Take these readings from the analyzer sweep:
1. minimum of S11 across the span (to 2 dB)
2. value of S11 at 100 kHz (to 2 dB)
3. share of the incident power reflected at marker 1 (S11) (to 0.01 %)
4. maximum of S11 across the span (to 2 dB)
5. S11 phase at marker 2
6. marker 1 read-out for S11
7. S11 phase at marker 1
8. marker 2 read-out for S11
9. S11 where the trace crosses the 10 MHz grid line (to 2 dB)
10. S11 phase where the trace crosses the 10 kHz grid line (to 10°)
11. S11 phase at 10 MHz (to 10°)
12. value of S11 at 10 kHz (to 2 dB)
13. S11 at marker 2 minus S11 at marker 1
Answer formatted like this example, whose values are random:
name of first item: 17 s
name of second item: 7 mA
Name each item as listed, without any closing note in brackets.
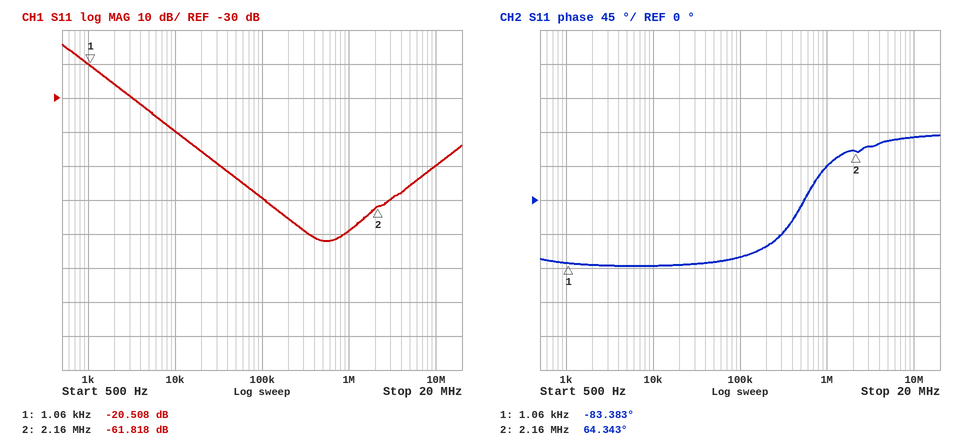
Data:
minimum of S11 across the span: -72 dB
value of S11 at 100 kHz: -60 dB
share of the incident power reflected at marker 1 (S11): 0.89 %
maximum of S11 across the span: -14 dB
S11 phase at marker 2: 64.343°
marker 1 read-out for S11: -20.508 dB
S11 phase at marker 1: -83.383°
marker 2 read-out for S11: -61.818 dB
S11 where the trace crosses the 10 MHz grid line: -50 dB
S11 phase where the trace crosses the 10 kHz grid line: -90°
S11 phase at 10 MHz: 80°
value of S11 at 10 kHz: -40 dB
S11 at marker 2 minus S11 at marker 1: -41.310 dB
